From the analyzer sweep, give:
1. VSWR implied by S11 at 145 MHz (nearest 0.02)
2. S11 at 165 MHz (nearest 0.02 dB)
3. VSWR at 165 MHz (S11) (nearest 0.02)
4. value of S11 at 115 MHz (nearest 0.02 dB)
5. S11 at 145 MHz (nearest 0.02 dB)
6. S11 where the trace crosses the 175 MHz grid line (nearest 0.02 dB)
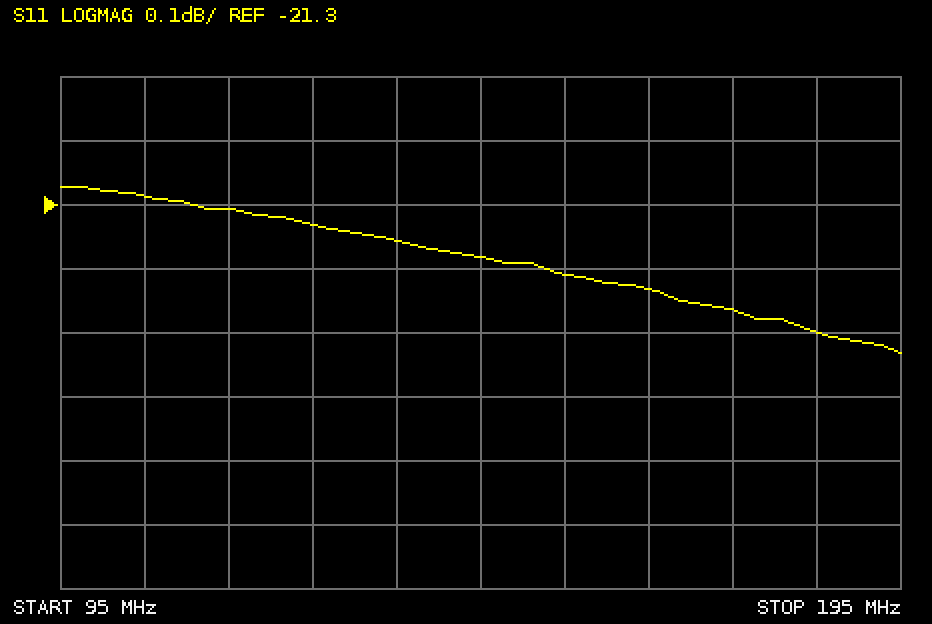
1.18
-21.44 dB
1.18
-21.30 dB
-21.38 dB
-21.46 dB
